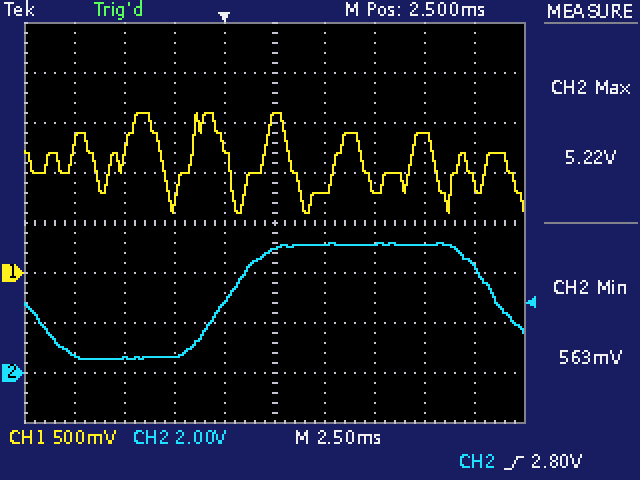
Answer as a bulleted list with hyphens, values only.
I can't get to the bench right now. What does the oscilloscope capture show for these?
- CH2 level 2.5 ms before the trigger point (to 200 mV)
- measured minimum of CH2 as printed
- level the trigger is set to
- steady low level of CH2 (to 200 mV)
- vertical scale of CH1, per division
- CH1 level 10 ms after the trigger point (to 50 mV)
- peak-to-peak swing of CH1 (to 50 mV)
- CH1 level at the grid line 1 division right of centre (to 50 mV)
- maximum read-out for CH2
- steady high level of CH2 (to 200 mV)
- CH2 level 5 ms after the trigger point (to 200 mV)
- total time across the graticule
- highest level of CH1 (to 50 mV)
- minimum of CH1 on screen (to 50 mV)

- 600 mV
- 563 mV
- 2.80 V
- 600 mV
- 500 mV
- 1.40 V
- 1.00 V
- 800 mV
- 5.22 V
- 5.2 V
- 5.2 V
- 25 ms
- 1.60 V
- 600 mV
